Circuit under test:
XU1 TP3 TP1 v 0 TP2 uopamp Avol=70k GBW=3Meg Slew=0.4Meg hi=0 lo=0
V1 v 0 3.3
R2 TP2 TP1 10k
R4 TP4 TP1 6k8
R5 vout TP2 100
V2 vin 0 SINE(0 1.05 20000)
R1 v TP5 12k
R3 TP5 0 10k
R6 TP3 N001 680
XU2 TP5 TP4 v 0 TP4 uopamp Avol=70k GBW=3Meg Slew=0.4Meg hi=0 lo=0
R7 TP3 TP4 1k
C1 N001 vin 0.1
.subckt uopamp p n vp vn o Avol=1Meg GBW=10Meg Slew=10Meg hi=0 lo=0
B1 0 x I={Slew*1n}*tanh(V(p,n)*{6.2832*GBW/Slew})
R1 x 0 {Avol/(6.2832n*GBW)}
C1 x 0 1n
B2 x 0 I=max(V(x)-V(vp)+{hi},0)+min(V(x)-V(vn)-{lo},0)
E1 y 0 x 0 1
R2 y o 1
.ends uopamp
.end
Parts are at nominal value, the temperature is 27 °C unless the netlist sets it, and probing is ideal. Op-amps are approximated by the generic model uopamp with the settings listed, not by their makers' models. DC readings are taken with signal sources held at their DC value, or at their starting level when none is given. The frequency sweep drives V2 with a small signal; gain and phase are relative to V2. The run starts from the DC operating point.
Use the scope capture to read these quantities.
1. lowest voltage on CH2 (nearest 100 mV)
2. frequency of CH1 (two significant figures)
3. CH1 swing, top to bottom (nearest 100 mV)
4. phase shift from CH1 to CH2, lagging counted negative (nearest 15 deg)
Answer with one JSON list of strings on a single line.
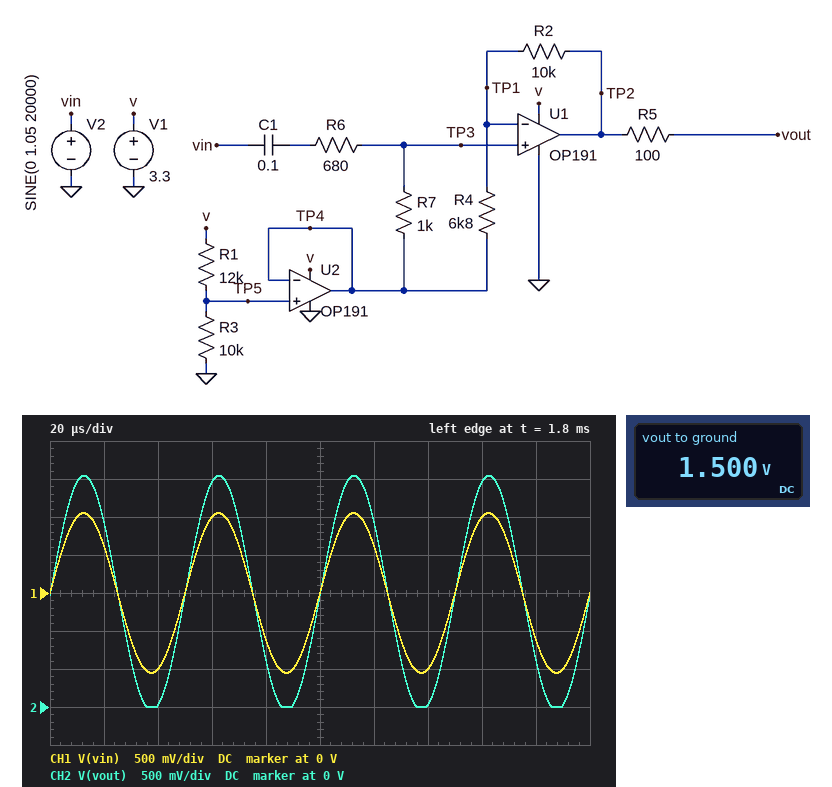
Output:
["0 V", "20 kHz", "2.1 V", "0 deg"]
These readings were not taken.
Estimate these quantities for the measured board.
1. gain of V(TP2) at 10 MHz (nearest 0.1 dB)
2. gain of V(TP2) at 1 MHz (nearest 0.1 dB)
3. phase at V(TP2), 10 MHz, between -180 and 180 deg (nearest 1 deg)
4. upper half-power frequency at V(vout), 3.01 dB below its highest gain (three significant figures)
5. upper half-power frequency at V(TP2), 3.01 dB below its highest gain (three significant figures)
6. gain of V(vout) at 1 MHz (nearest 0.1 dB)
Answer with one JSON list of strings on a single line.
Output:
["-15.0 dB", "1.1 dB", "-83 deg", "1.21 MHz", "1.21 MHz", "1.1 dB"]
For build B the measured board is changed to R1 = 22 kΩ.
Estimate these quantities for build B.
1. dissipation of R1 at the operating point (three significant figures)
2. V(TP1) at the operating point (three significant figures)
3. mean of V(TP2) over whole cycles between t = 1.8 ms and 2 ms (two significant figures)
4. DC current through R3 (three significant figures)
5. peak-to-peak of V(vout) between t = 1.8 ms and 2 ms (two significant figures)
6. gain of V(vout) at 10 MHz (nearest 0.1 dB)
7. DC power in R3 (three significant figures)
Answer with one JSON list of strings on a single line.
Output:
["234 µW", "1.03 V", "1.1 V", "103 µA", "2.6 V", "-15.0 dB", "106 µW"]
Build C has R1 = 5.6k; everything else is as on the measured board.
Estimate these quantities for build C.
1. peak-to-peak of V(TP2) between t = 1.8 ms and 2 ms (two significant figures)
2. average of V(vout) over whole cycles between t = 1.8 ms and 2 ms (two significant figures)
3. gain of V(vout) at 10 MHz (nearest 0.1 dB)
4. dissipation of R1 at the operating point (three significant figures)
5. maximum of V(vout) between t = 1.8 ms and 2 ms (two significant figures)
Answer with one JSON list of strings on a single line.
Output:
["2.7 V", "2.1 V", "-15.0 dB", "251 µW", "3.3 V"]
